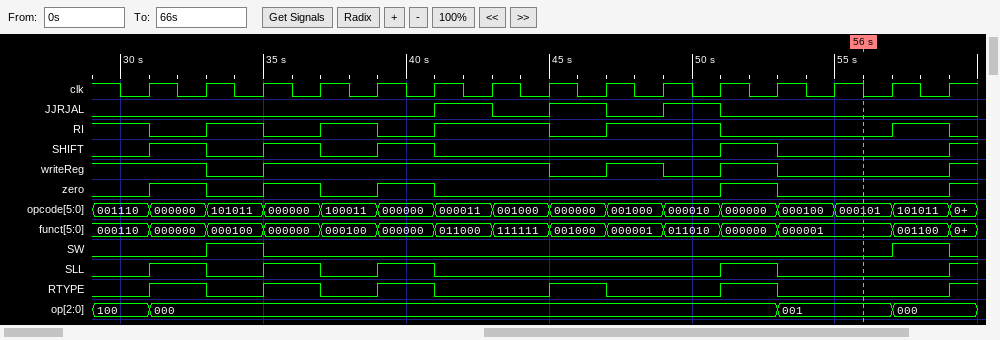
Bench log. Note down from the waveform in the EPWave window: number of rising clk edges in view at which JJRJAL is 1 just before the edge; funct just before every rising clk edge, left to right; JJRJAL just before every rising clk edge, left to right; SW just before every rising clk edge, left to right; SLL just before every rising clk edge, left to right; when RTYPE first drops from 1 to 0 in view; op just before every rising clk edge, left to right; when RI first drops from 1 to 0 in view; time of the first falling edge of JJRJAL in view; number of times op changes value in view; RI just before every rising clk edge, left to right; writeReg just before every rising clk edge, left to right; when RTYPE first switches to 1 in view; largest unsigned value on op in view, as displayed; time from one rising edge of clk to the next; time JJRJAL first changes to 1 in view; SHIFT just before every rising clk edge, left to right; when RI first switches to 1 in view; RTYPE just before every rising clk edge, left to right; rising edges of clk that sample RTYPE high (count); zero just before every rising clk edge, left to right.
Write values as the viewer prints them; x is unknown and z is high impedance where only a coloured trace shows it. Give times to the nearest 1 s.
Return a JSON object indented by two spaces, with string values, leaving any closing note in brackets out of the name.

{
  "number of rising clk edges in view at which JJRJAL is 1 just before the edge": "3",
  "funct just before every rising clk edge, left to right": "000110, 000000, 000100, 000000, 000100, 000000, 011000, 111111, 001000, 000001, 011010, 000000, 000001, 000001, 001100",
  "JJRJAL just before every rising clk edge, left to right": "0 0 0 0 0 0 1 0 1 0 1 0 0 0 0",
  "SW just before every rising clk edge, left to right": "0 0 1 0 0 0 0 0 0 0 0 0 0 0 1",
  "SLL just before every rising clk edge, left to right": "0 1 0 1 0 1 0 0 0 0 0 1 0 0 0",
  "when RTYPE first drops from 1 to 0 in view": "33 s",
  "op just before every rising clk edge, left to right": "100, 000, 000, 000, 000, 000, 000, 000, 000, 000, 000, 000, 001, 001, 000",
  "when RI first drops from 1 to 0 in view": "31 s",
  "time of the first falling edge of JJRJAL in view": "43 s",
  "number of times op changes value in view": "3",
  "RI just before every rising clk edge, left to right": "1 0 1 0 1 0 1 1 0 1 1 0 0 0 1",
  "writeReg just before every rising clk edge, left to right": "1 1 0 1 1 1 1 1 0 1 0 1 0 0 0",
  "when RTYPE first switches to 1 in view": "31 s",
  "largest unsigned value on op in view, as displayed": "100",
  "time from one rising edge of clk to the next": "2 s",
  "time JJRJAL first changes to 1 in view": "41 s",
  "SHIFT just before every rising clk edge, left to right": "0 1 0 1 0 1 0 0 0 0 0 1 0 0 0",
  "when RI first switches to 1 in view": "33 s",
  "RTYPE just before every rising clk edge, left to right": "0 1 0 1 0 1 0 0 1 0 0 1 0 0 0",
  "rising edges of clk that sample RTYPE high": "5",
  "zero just before every rising clk edge, left to right": "0 1 0 1 0 1 0 0 0 0 0 1 0 0 0"
}
